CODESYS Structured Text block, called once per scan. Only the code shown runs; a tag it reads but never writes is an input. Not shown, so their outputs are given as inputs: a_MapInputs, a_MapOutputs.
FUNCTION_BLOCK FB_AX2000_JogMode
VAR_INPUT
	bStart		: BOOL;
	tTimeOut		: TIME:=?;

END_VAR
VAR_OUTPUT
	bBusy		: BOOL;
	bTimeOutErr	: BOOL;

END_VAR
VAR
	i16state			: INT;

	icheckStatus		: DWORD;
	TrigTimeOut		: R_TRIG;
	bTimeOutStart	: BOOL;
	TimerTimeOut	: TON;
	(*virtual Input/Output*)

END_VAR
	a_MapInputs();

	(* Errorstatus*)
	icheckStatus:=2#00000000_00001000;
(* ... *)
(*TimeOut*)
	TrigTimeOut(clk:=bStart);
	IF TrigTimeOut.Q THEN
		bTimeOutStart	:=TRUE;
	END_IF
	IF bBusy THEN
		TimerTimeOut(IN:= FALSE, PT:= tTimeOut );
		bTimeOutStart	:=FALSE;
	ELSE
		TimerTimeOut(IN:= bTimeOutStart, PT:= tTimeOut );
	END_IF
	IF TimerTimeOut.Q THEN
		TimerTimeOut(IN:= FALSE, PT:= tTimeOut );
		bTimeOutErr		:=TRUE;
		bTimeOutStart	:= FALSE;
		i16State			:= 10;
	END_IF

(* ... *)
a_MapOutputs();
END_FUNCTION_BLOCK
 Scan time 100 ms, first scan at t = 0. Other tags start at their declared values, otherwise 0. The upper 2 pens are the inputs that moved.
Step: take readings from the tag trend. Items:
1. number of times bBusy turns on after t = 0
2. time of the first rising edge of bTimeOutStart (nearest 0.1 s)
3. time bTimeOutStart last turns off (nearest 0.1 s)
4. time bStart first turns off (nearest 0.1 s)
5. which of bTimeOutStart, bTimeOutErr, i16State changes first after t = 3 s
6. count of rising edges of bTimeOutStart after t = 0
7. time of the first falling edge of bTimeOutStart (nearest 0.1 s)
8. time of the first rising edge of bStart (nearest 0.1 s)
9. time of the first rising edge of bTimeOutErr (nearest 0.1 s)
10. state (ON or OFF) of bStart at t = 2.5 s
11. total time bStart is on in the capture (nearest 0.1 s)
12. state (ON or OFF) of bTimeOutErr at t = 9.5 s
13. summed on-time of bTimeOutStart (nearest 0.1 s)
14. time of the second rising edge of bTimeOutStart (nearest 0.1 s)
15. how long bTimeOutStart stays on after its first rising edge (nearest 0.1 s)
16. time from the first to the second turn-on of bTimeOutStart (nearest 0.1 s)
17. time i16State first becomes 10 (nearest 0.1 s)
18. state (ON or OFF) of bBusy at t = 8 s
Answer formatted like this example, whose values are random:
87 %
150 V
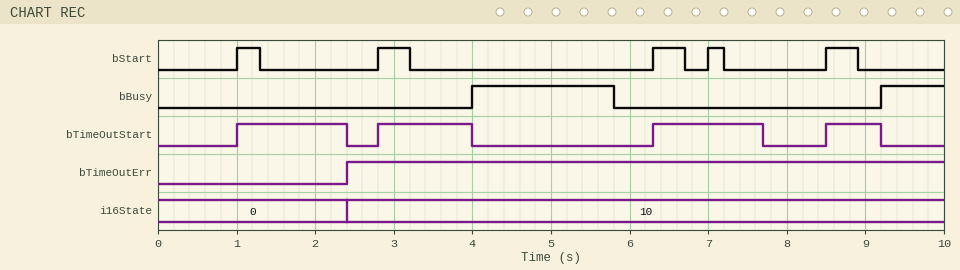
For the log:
2
1.0 s
9.2 s
1.3 s
bTimeOutStart
4
2.4 s
1.0 s
2.4 s
OFF
1.7 s
ON
4.7 s
2.8 s
1.4 s
1.8 s
2.4 s
OFF
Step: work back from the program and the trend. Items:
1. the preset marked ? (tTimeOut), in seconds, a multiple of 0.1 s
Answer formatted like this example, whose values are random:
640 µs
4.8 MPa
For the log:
1.4 s
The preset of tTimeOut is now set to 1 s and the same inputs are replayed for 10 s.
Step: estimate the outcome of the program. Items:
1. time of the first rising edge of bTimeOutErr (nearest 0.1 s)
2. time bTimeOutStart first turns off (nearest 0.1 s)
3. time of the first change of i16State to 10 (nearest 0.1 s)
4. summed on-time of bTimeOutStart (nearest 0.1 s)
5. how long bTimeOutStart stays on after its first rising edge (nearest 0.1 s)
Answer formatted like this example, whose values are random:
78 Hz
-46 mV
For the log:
2.0 s
2.0 s
2.0 s
3.7 s
1.0 s
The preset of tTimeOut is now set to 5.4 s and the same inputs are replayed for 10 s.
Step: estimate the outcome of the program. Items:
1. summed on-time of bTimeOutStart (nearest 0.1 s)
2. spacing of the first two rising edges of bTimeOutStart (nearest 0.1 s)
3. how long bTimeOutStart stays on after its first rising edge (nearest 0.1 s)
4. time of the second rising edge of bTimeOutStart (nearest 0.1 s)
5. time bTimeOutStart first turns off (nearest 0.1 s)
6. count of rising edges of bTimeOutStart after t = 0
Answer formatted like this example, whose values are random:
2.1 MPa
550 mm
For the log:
5.9 s
5.3 s
3.0 s
6.3 s
4.0 s
2
